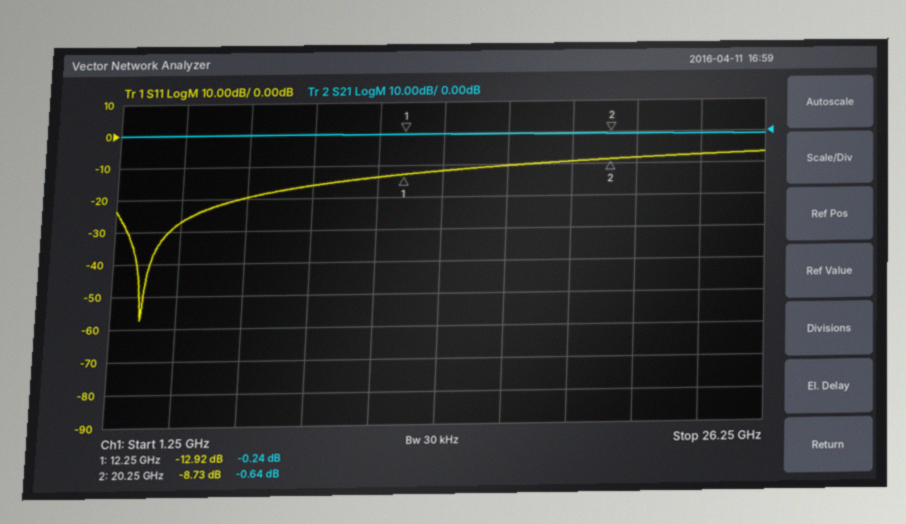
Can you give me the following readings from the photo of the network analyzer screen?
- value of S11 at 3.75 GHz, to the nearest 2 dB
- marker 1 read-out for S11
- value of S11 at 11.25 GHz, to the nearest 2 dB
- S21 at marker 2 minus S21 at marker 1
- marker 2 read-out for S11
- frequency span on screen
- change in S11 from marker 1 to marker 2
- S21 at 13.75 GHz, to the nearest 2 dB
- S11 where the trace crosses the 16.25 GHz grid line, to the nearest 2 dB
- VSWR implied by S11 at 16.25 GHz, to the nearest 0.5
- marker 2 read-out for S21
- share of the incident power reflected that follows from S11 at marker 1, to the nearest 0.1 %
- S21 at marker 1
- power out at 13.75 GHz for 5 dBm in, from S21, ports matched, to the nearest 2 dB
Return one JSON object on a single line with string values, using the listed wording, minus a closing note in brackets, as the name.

{"value of S11 at 3.75 GHz, to the nearest 2 dB": "-28 dB", "marker 1 read-out for S11": "-12.92 dB", "value of S11 at 11.25 GHz, to the nearest 2 dB": "-14 dB", "S21 at marker 2 minus S21 at marker 1": "-0.40 dB", "marker 2 read-out for S11": "-8.73 dB", "frequency span on screen": "25 GHz", "change in S11 from marker 1 to marker 2": "4.19 dB", "S21 at 13.75 GHz, to the nearest 2 dB": "0 dB", "S11 where the trace crosses the 16.25 GHz grid line, to the nearest 2 dB": "-10 dB", "VSWR implied by S11 at 16.25 GHz, to the nearest 0.5": "2.0", "marker 2 read-out for S21": "-0.64 dB", "share of the incident power reflected that follows from S11 at marker 1, to the nearest 0.1 %": "5.1 %", "S21 at marker 1": "-0.24 dB", "power out at 13.75 GHz for 5 dBm in, from S21, ports matched, to the nearest 2 dB": "4 dBm"}
